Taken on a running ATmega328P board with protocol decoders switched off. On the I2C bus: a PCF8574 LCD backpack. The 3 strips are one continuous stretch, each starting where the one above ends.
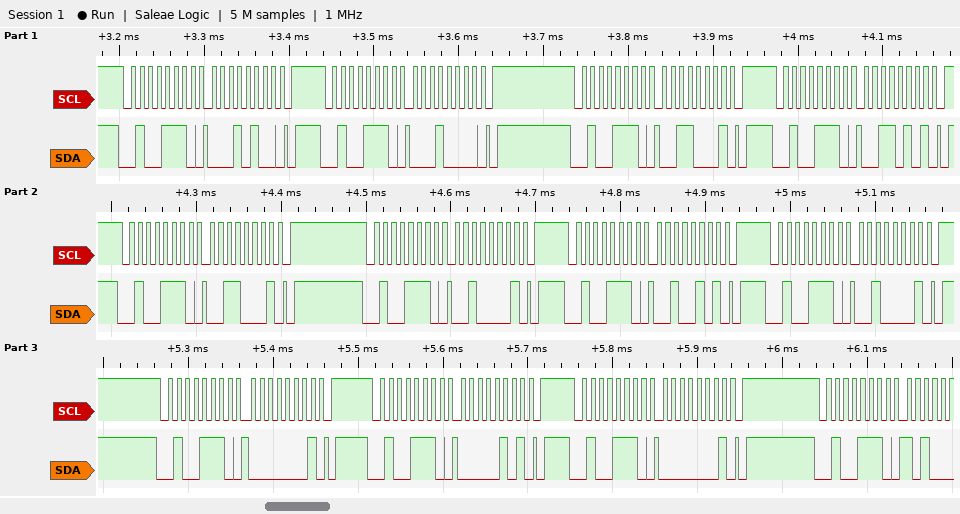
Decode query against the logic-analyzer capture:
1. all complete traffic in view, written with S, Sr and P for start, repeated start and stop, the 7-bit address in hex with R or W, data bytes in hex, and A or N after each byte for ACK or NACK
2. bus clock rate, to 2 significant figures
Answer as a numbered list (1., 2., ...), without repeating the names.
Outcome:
1. S 27W A 14 A P S 27W A 10 A P S 27W A 31 A P S 27W A 35 A P S 27W A 31 A P S 27W A 21 A P S 27W A 25 A P S 27W A 21 A P S 27W A 01 A P S 27W A 05 A P S 27W A 01 A P S 27W A
2. 100 kHz
